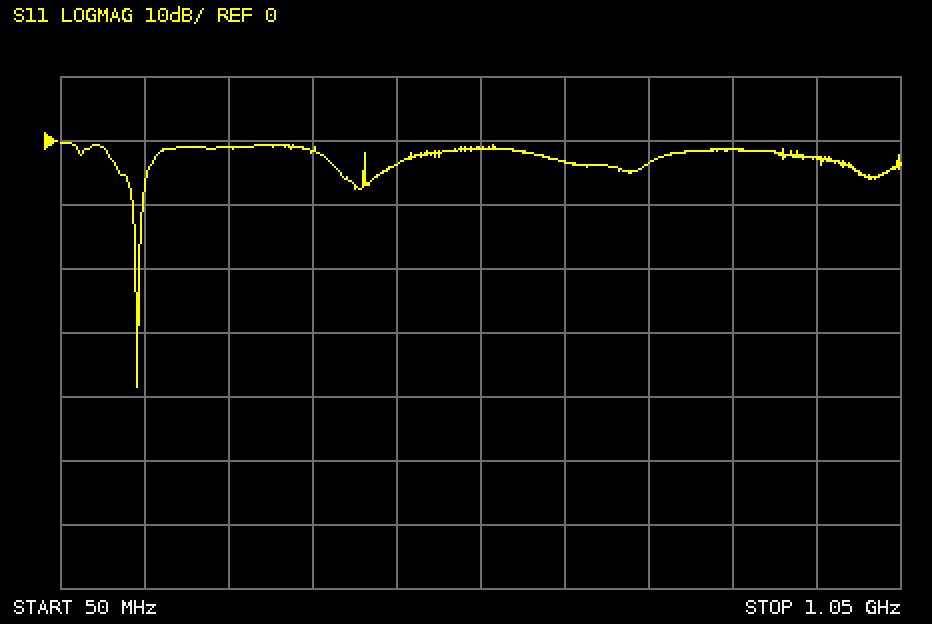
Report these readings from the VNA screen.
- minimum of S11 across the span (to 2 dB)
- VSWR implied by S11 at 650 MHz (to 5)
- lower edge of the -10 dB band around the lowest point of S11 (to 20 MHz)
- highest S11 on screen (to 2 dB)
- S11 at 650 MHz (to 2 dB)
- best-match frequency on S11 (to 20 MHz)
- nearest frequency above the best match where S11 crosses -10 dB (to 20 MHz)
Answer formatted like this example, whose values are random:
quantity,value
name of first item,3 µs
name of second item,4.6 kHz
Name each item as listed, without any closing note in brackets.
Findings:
quantity,value
minimum of S11 across the span,-38 dB
VSWR implied by S11 at 650 MHz,5
lower edge of the -10 dB band around the lowest point of S11,140 MHz
highest S11 on screen,0 dB
S11 at 650 MHz,-4 dB
best-match frequency on S11,140 MHz
nearest frequency above the best match where S11 crosses -10 dB,140 MHz
